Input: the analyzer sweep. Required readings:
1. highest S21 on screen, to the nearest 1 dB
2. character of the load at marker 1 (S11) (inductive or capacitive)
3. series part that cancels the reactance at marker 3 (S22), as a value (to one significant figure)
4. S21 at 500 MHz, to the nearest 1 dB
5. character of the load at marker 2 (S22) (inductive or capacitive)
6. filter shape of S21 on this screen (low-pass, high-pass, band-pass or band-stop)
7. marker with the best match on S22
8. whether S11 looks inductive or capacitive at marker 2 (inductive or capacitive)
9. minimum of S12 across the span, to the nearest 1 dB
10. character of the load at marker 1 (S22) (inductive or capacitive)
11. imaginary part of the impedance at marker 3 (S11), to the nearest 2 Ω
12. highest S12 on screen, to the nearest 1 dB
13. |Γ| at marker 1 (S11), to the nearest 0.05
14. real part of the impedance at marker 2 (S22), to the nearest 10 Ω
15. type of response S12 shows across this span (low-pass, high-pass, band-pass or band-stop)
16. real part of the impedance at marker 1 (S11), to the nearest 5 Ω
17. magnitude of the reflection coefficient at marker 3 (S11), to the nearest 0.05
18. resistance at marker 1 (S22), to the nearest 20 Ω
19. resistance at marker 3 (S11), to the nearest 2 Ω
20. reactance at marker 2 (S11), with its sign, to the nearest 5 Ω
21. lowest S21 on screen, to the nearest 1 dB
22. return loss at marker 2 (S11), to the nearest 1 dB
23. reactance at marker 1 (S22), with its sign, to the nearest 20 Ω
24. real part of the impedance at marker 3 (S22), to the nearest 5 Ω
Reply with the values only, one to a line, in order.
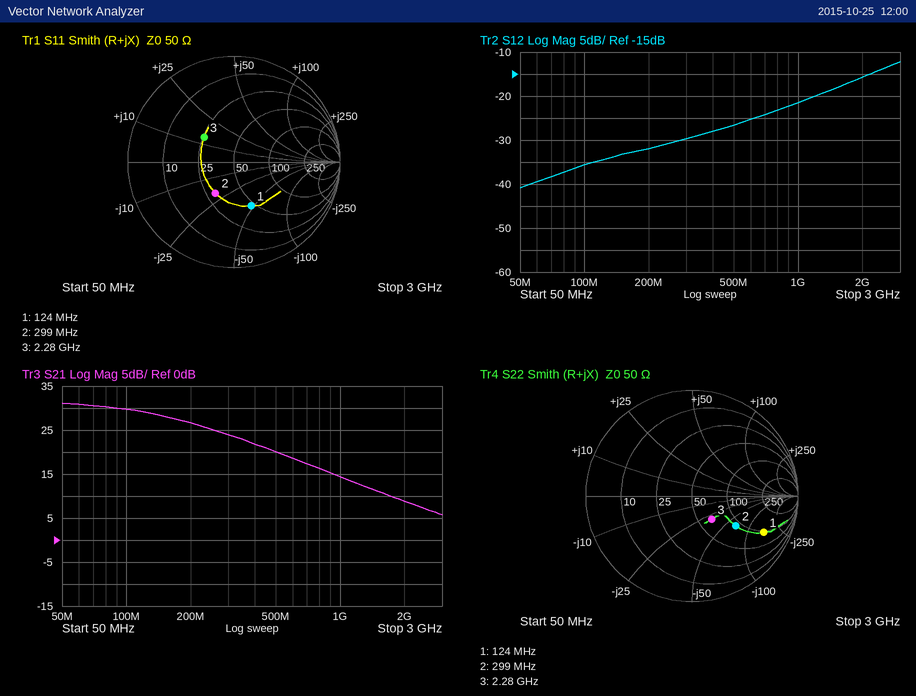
31 dB
capacitive
2 nH
20 dB
capacitive
low-pass
marker 3
capacitive
-41 dB
capacitive
+14 Ω
-12 dB
0.45
90 Ω
high-pass
45 Ω
0.35
100 Ω
26 Ω
-20 Ω
6 dB
9 dB
-160 Ω
65 Ω
